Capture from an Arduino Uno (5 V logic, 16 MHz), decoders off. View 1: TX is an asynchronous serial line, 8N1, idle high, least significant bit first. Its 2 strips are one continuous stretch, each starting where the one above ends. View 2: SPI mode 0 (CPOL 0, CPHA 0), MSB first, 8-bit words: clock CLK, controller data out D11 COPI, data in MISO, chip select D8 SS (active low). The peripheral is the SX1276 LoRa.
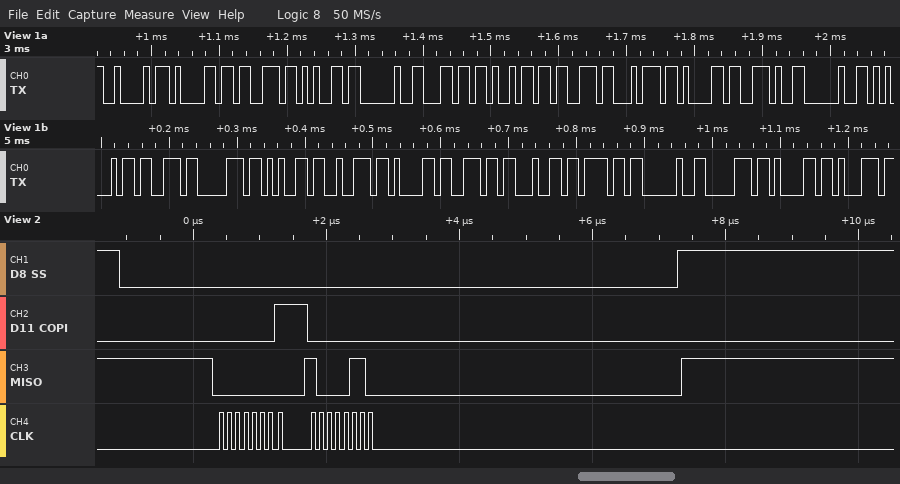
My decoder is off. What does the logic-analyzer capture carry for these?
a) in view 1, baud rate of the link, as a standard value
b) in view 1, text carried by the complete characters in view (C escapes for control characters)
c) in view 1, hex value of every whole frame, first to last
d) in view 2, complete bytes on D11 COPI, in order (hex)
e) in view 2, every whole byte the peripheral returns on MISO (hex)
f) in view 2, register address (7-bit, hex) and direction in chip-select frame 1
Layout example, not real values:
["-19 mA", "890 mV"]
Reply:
["115200 baud", "\"Base lista. Esperando paq\"", "42 61 73 65 20 6C 69 73 74 61 2E 20 45 73 70 65 72 61 6E 64 6F 20 70 61 71", "01 00", "00 86", "0x01 read"]
